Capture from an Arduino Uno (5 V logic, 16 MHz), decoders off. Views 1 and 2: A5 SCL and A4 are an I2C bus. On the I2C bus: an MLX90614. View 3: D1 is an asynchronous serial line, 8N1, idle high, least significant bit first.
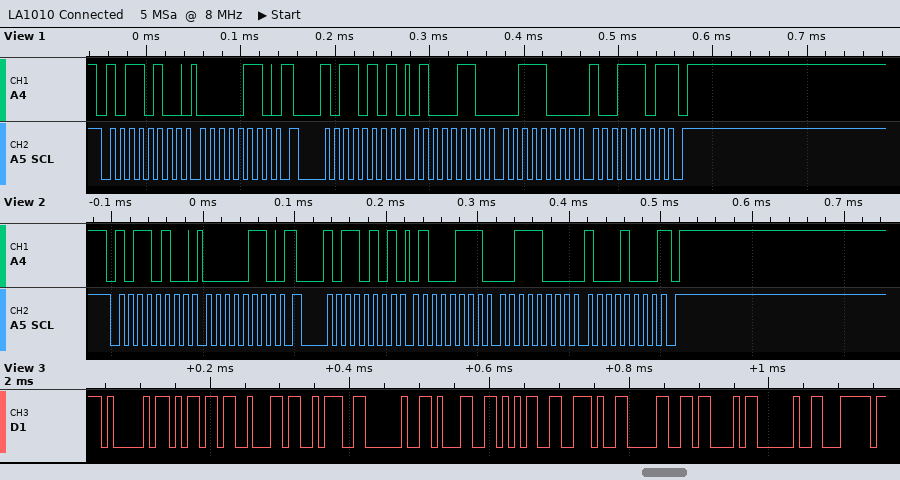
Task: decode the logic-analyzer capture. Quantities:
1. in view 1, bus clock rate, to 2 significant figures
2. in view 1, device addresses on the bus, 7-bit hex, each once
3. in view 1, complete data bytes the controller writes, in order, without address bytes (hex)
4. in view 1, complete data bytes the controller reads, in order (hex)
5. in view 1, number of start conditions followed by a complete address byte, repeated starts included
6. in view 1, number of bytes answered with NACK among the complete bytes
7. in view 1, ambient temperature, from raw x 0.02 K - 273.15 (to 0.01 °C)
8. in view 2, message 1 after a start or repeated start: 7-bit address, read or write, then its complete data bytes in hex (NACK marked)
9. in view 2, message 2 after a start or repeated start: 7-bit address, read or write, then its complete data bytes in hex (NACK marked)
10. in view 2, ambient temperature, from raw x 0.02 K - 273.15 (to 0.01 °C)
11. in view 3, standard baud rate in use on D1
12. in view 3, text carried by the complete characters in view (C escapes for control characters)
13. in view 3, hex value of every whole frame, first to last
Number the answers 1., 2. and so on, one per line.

1. 100 kHz
2. 0x5A
3. 06
4. 46 38 9D
5. 2
6. 1
7. 14.97 °C
8. 0x5A write: 06
9. 0x5A read: 47 38 88 NACK
10. 14.99 °C
11. 115200 baud
12. "Amb: 15.0C |"
13. 41 6D 62 3A 20 31 35 2E 30 43 20 7C
